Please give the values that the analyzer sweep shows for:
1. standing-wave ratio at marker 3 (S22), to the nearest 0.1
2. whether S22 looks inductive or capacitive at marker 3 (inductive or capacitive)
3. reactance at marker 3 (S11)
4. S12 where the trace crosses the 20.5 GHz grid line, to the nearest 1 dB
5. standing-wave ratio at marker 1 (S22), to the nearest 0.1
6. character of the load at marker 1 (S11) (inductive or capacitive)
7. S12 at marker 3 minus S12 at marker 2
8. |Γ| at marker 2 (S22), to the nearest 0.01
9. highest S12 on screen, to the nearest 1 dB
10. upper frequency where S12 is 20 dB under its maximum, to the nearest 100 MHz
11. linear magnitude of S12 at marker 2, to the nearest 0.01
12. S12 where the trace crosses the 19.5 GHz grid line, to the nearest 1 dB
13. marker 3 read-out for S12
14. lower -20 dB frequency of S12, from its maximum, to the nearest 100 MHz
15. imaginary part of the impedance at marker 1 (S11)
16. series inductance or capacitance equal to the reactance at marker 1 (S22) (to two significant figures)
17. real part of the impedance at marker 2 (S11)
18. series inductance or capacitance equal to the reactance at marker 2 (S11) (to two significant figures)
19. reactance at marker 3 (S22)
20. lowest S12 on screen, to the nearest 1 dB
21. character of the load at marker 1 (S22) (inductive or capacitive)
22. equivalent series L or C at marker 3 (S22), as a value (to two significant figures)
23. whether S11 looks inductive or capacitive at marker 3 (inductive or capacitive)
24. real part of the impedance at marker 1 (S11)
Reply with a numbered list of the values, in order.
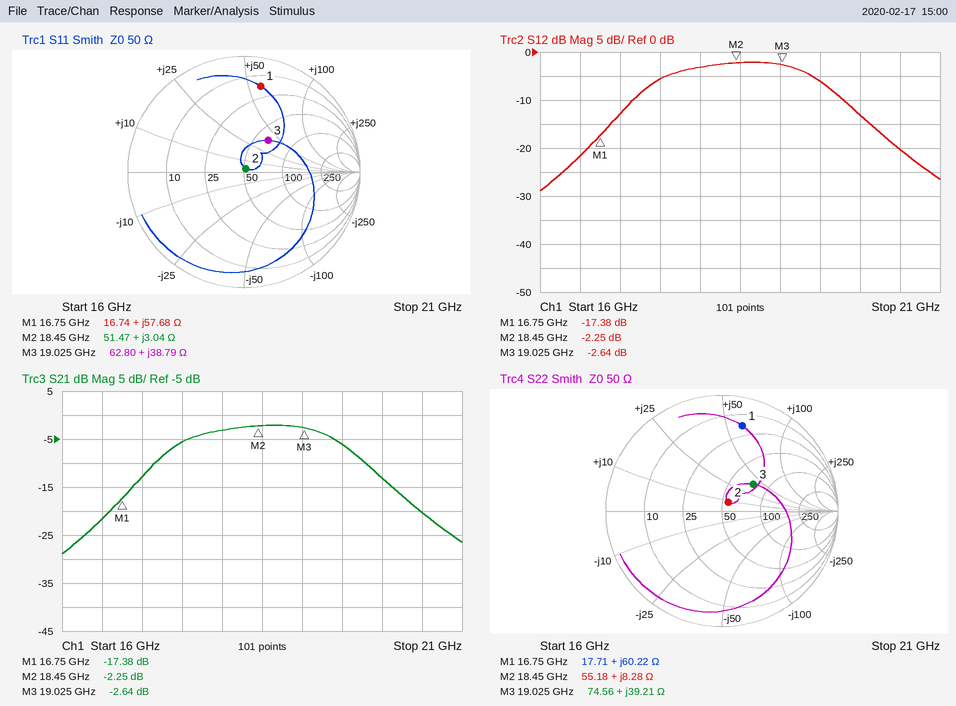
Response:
1. 2.1
2. inductive
3. +38.79 Ω
4. -20 dB
5. 7.1
6. inductive
7. -0.39 dB
8. 0.09
9. -2 dB
10. 20.6 GHz
11. 0.77
12. -6 dB
13. -2.64 dB
14. 16.5 GHz
15. +57.68 Ω
16. 570 pH
17. 51.47 Ω
18. 26 pH
19. +39.21 Ω
20. -29 dB
21. inductive
22. 330 pH
23. inductive
24. 16.74 Ω
